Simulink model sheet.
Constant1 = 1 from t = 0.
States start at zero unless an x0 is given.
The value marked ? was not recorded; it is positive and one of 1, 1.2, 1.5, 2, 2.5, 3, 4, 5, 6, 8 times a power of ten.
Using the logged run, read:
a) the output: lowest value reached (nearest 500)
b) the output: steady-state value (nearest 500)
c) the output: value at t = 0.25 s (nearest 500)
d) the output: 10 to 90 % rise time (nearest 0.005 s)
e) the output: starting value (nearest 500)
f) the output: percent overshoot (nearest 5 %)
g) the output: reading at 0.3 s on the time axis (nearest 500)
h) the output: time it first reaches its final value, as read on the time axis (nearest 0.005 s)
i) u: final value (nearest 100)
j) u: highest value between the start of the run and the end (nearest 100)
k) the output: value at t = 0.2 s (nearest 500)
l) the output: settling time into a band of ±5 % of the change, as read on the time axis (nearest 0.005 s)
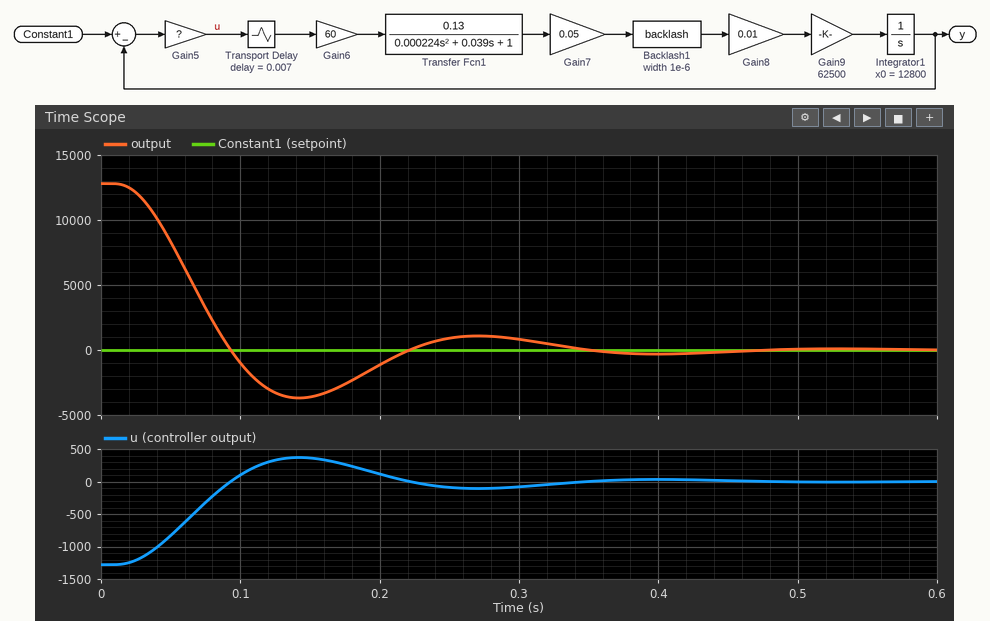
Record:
-3500
0
1000
0.055 s
13000
30 %
1000
0.095 s
0
400
-1000
0.310 s
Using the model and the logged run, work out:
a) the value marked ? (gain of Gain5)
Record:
0.1
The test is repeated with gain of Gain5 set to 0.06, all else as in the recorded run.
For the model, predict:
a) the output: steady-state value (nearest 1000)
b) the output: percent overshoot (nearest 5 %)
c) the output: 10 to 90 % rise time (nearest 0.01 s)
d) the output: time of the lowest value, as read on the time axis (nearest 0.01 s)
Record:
0
10 %
0.09 s
0.20 s
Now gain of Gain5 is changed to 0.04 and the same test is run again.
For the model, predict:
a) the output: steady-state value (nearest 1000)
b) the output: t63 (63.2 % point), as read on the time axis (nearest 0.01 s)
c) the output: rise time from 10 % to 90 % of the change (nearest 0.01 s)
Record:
0
0.12 s
0.14 s
